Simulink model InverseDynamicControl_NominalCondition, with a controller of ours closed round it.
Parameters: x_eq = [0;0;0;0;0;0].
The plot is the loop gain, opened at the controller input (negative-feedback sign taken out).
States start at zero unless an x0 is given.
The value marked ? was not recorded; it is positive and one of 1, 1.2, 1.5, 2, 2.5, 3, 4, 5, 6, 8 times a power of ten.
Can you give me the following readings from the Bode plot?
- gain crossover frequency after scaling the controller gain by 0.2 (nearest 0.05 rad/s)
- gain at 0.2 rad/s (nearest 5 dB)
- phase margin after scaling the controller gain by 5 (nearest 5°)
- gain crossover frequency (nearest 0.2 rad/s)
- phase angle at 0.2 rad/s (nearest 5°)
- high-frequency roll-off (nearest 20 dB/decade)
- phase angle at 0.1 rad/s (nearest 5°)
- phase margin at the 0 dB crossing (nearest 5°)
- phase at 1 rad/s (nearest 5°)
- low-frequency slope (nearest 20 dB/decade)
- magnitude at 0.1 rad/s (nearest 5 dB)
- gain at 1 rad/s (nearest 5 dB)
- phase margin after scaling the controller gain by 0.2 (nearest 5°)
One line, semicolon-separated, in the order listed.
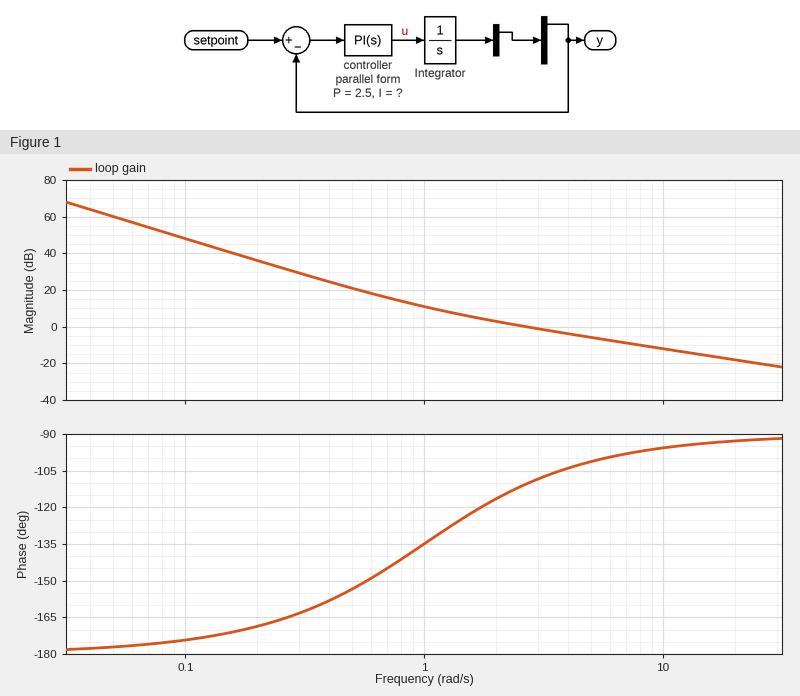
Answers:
0.80 rad/s; 35 dB; 85°; 2.6 rad/s; -170°; -20 dB/decade; -175°; 70°; -135°; -40 dB/decade; 50 dB; 10 dB; 40°
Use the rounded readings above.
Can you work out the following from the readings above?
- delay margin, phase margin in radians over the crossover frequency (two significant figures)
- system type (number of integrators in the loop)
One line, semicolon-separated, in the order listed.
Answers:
0.47 s; 2
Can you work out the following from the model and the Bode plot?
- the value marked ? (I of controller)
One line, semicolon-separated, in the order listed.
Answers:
2.5
